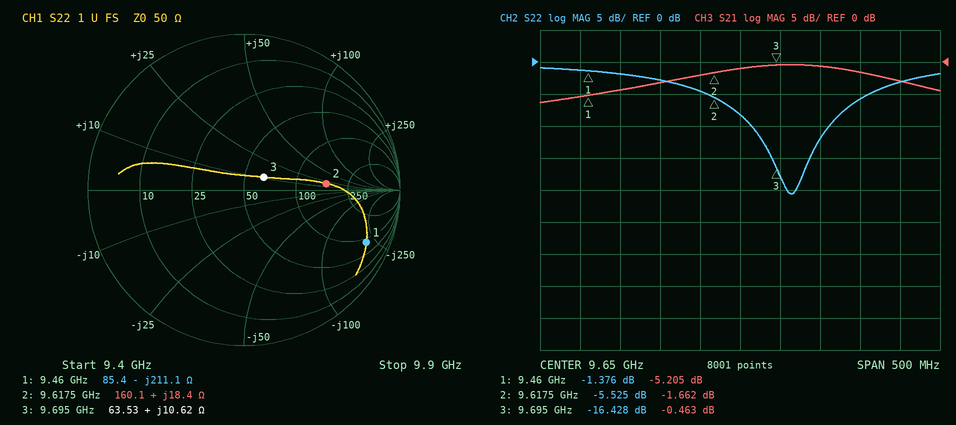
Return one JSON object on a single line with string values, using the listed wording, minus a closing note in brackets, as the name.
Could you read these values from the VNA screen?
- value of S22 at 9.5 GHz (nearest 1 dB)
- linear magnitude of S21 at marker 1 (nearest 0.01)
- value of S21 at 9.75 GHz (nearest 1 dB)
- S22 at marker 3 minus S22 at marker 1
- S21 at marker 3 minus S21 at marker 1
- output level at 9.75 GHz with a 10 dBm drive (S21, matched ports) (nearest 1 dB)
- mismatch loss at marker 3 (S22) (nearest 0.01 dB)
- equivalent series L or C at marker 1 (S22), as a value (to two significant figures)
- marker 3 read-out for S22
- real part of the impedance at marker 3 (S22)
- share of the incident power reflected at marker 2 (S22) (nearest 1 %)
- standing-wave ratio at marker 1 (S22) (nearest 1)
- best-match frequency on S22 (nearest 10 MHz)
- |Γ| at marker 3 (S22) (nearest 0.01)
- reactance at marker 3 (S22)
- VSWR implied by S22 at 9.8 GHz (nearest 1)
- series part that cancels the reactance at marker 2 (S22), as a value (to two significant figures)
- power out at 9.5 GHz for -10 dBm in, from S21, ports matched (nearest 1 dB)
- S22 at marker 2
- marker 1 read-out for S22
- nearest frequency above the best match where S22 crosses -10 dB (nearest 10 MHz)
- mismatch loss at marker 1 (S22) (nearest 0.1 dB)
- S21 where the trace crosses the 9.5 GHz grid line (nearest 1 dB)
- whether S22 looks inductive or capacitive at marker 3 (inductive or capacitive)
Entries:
{"value of S22 at 9.5 GHz": "-2 dB", "linear magnitude of S21 at marker 1": "0.55", "value of S21 at 9.75 GHz": "-1 dB", "S22 at marker 3 minus S22 at marker 1": "-15.052 dB", "S21 at marker 3 minus S21 at marker 1": "4.742 dB", "output level at 9.75 GHz with a 10 dBm drive (S21, matched ports)": "9 dBm", "mismatch loss at marker 3 (S22)": "0.10 dB", "equivalent series L or C at marker 1 (S22), as a value": "80 fF", "marker 3 read-out for S22": "-16.428 dB", "real part of the impedance at marker 3": "63.53 Ω", "share of the incident power reflected at marker 2 (S22)": "28 %", "standing-wave ratio at marker 1 (S22)": "13", "best-match frequency on S22": "9.71 GHz", "|Γ| at marker 3 (S22)": "0.15", "reactance at marker 3": "+10.62 Ω", "VSWR implied by S22 at 9.8 GHz": "3", "series part that cancels the reactance at marker 2 (S22), as a value": "900 fF", "power out at 9.5 GHz for -10 dBm in, from S21, ports matched": "-14 dBm", "S22 at marker 2": "-5.525 dB", "marker 1 read-out for S22": "-1.376 dB", "nearest frequency above the best match where S22 crosses -10 dB": "9.76 GHz", "mismatch loss at marker 1 (S22)": "5.7 dB", "S21 where the trace crosses the 9.5 GHz grid line": "-4 dB", "whether S22 looks inductive or capacitive at marker 3": "inductive"}
